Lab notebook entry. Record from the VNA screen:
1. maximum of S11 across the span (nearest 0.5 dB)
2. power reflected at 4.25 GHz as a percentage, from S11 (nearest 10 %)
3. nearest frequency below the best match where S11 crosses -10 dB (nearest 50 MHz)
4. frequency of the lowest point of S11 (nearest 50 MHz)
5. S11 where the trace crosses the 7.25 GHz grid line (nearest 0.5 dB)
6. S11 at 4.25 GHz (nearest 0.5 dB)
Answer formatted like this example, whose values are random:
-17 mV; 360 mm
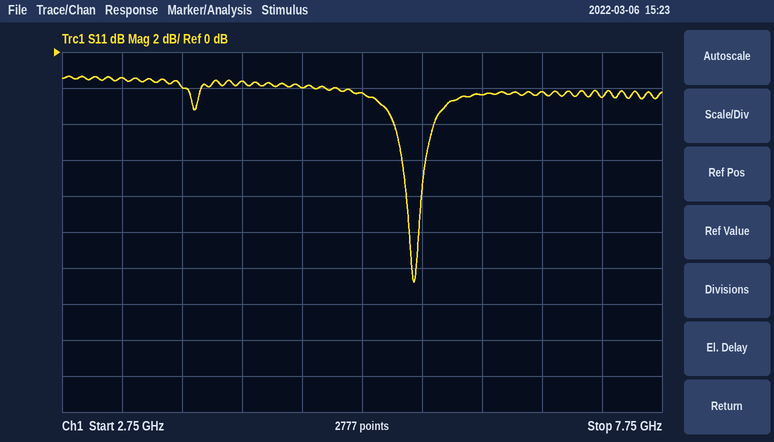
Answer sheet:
-1.5 dB; 70 %; 5.65 GHz; 5.70 GHz; -2.5 dB; -1.5 dB
